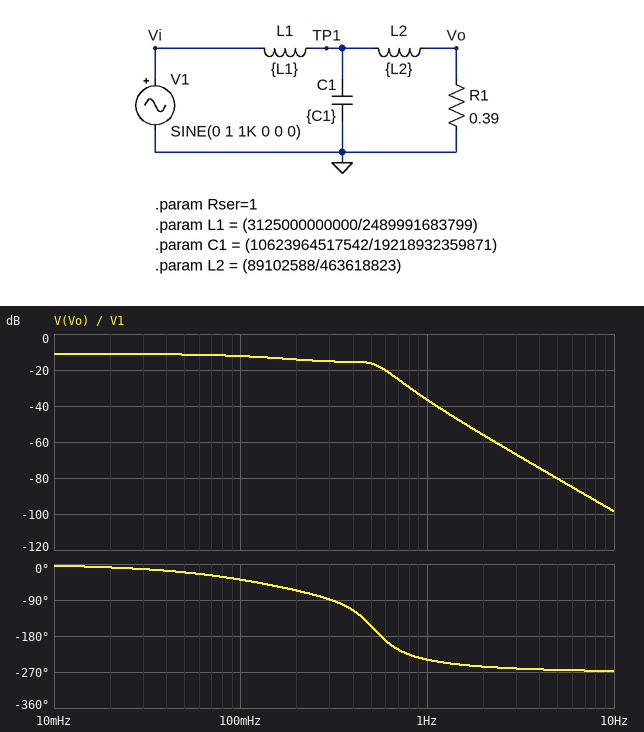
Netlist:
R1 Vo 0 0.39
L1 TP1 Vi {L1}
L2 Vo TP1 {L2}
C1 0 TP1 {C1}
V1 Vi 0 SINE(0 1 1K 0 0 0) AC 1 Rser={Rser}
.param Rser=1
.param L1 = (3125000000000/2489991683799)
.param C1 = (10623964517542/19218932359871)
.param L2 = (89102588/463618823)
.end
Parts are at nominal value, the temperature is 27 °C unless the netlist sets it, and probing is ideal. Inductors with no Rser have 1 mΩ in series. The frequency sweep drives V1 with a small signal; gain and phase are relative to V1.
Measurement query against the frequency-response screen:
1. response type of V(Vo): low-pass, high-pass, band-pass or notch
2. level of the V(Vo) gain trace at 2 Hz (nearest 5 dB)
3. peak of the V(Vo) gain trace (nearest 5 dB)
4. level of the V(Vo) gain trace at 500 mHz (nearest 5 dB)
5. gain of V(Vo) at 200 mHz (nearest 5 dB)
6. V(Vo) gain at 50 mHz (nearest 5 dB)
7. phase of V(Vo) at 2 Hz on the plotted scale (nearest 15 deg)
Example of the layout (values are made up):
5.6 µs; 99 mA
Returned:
low-pass; -55 dB; -10 dB; -15 dB; -15 dB; -10 dB; -255 deg
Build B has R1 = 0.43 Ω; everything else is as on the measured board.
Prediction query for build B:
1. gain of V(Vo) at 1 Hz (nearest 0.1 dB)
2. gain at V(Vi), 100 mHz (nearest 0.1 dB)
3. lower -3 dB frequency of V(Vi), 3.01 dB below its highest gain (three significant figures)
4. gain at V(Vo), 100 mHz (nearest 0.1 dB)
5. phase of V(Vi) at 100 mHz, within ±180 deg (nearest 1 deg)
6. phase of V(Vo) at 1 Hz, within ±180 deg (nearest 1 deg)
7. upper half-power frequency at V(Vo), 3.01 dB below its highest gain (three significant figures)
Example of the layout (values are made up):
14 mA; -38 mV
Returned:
-35.9 dB; -4.9 dB; 158 mHz; -11.6 dB; 31 deg; 123 deg; 203 mHz
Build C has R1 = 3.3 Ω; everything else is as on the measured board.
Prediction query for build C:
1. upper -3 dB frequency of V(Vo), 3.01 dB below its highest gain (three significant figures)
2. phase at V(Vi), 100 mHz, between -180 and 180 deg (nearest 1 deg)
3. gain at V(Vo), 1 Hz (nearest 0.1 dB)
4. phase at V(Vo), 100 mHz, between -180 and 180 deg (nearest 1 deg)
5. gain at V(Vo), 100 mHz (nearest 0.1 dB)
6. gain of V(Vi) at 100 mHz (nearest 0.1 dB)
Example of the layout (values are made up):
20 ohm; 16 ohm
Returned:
260 mHz; -11 deg; -28.8 dB; -31 deg; -1.5 dB; -3.7 dB
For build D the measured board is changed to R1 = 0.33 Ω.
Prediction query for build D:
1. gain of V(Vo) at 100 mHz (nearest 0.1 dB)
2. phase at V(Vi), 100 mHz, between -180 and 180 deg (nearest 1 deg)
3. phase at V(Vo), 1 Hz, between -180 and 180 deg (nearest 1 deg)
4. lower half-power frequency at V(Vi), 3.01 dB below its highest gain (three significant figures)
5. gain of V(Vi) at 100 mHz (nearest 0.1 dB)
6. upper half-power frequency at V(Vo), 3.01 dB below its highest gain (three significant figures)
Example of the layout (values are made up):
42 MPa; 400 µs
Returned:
-13.5 dB; 35 deg; 118 deg; 146 mHz; -4.7 dB; 181 mHz
